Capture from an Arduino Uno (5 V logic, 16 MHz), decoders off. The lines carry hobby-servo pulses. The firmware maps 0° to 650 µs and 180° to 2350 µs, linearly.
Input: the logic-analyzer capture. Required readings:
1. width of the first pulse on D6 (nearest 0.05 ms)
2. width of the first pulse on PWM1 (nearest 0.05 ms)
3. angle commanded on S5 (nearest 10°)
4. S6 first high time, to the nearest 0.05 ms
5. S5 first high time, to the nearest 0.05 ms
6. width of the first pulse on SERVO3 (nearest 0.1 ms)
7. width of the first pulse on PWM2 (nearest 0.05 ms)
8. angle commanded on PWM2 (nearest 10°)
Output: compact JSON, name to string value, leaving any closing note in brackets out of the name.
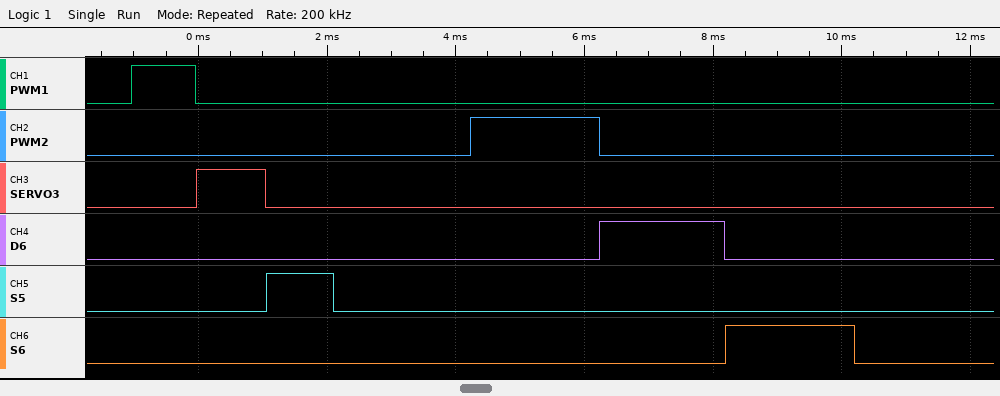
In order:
{"width of the first pulse on D6": "1.95 ms", "width of the first pulse on PWM1": "1.00 ms", "angle commanded on S5": "40°", "S6 first high time, to the nearest 0.05 ms": "2.00 ms", "S5 first high time, to the nearest 0.05 ms": "1.05 ms", "width of the first pulse on SERVO3": "1.1 ms", "width of the first pulse on PWM2": "2.00 ms", "angle commanded on PWM2": "140°"}
